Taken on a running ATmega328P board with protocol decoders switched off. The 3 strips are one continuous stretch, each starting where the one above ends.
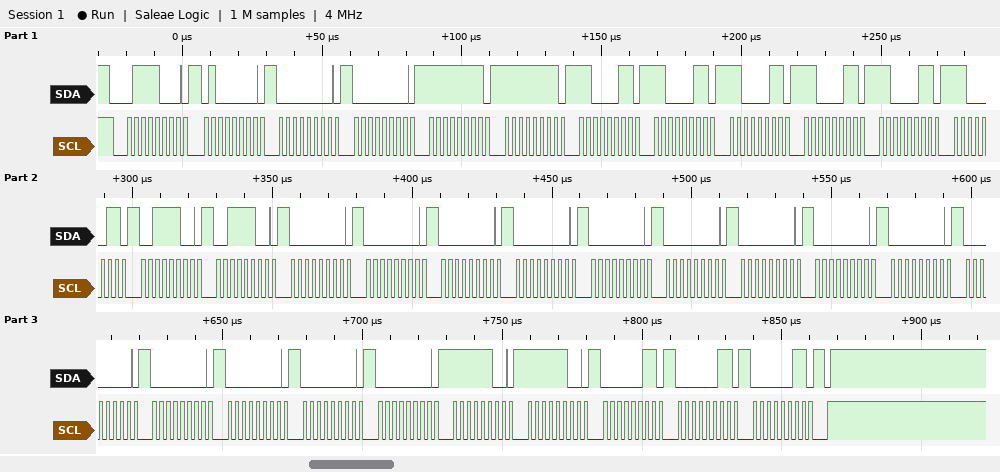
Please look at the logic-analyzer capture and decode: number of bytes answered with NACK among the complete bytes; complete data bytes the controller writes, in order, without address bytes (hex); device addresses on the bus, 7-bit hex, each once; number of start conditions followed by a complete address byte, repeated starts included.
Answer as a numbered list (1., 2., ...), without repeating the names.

1. 0
2. 40 00 00 FF FF C3 C3 C3 C3 C3 C3 3C 3C 00 00 00 00 00 00 00 00 00 00 00 00 00 00 FC FC 03 03 03
3. 0x3C
4. 1
